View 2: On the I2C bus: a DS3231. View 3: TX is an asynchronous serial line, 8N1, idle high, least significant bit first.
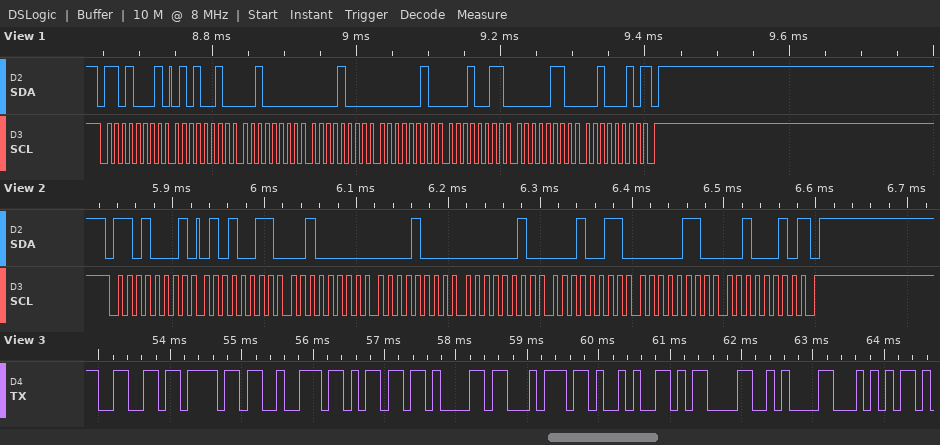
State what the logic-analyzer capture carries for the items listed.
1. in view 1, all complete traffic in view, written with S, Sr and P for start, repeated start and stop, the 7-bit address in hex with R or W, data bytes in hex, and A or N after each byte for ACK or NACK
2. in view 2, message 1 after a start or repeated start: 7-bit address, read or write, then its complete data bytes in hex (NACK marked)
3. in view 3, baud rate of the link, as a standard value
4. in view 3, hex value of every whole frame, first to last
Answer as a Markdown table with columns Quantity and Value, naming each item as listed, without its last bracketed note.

| Quantity | Value |
|---|---|
| in view 1, all complete traffic in view, written with S, Sr and P for start, repeated start and stop, the 7-bit address in hex with R or W, data bytes in hex, and A or N after each byte for ACK or NACK | S 68R A 52 A 20 A 08 A 02 A 13 A 06 A 22 N P |
| in view 2, message 1 after a start or repeated start: 7-bit address, read or write, then its complete data bytes in hex | 0x68 read: 53 20 08 02 13 06 22 NACK |
| in view 3, baud rate of the link, as a standard value | 9600 baud |
| in view 3, hex value of every whole frame, first to last | 0x66 0x6F 0x72 0x6D 0x61 0x74 0x29 0x0D 0x0A 0x54 |
